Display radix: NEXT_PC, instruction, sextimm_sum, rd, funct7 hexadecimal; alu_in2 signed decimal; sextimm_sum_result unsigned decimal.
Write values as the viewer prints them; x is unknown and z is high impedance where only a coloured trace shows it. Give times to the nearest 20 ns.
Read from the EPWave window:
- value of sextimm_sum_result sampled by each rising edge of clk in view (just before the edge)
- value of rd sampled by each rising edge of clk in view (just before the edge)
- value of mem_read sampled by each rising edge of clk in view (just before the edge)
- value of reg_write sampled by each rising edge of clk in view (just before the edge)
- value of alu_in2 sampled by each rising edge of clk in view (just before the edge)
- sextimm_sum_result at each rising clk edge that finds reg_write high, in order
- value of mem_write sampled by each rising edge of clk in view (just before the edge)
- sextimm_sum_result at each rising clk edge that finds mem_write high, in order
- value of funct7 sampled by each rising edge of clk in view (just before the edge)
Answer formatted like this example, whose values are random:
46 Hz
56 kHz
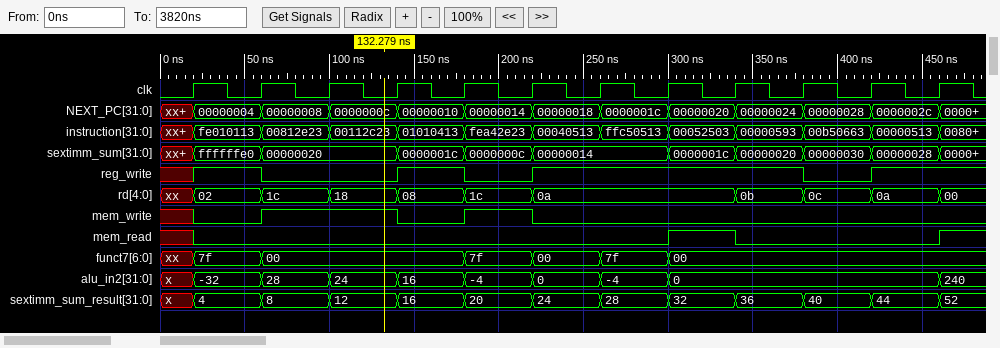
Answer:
x, 4, 8, 12, 16, 20, 24, 28, 32, 36, 40, 44
xx, 02, 1c, 18, 08, 1c, 0a, 0a, 0a, 0b, 0c, 0a
x 0 0 0 0 0 0 0 1 0 0 0
x 1 0 0 1 0 1 1 1 1 0 1
x, -32, 28, 24, 16, -4, 0, -4, 0, 0, 0, 0
4, 16, 24, 28, 32, 36, 44
x 0 1 1 0 1 0 0 0 0 0 0
8, 12, 20
xx, 7f, 00, 00, 00, 7f, 00, 7f, 00, 00, 00, 00
